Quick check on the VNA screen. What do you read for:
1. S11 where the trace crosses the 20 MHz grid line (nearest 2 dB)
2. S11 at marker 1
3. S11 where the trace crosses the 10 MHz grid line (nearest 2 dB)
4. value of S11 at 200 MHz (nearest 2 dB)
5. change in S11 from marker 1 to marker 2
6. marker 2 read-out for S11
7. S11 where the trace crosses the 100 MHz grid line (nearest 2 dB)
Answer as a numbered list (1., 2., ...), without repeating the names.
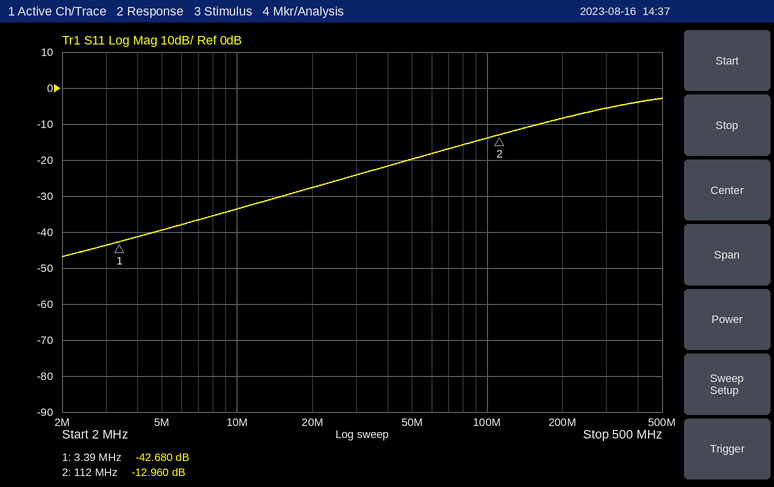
1. -28 dB
2. -42.680 dB
3. -34 dB
4. -8 dB
5. 29.720 dB
6. -12.960 dB
7. -14 dB
